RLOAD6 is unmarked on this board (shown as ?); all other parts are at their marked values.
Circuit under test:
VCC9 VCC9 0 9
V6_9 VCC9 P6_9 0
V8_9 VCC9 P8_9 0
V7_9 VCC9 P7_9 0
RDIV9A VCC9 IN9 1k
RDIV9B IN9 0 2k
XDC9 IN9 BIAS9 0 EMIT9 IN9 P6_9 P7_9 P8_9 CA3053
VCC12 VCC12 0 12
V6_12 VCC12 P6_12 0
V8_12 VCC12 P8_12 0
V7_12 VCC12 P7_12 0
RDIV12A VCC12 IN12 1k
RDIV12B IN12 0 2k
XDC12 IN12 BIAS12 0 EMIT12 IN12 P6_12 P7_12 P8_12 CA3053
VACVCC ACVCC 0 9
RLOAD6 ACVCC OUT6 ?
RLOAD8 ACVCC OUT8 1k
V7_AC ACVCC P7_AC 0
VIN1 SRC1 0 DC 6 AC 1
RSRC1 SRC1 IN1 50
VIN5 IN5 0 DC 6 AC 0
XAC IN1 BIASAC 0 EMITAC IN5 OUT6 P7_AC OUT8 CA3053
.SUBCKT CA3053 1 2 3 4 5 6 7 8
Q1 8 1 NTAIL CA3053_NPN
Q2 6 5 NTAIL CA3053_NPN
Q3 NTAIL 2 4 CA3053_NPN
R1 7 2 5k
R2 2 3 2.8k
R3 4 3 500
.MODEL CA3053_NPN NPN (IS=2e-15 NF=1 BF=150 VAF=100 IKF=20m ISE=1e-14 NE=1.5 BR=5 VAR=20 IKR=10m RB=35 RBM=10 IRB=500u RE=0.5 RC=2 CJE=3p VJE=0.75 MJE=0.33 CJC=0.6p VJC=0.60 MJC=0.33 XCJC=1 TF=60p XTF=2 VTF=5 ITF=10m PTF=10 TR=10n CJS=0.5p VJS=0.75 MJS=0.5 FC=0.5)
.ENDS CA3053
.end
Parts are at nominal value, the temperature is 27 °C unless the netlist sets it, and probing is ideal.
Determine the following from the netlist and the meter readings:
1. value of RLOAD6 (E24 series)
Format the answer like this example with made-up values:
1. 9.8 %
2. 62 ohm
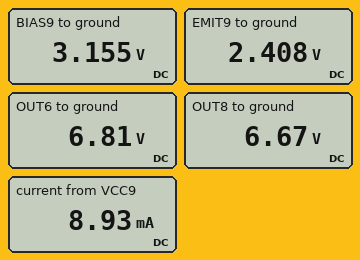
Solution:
1. 910 Ω
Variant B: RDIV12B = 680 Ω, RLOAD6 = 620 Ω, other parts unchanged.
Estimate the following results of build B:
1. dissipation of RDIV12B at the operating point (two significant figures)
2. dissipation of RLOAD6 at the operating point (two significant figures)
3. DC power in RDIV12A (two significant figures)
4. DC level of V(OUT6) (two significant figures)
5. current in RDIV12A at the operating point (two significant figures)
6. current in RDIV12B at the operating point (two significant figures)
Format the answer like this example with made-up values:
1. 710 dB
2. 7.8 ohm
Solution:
1. 34 mW
2. 3.6 mW
3. 51 mW
4. 7.5 V
5. 7.2 mA
6. 7.1 mA
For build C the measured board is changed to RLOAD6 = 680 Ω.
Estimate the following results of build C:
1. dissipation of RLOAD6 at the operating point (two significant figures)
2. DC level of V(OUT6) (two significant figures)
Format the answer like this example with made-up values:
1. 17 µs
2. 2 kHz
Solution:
1. 4.0 mW
2. 7.4 V
